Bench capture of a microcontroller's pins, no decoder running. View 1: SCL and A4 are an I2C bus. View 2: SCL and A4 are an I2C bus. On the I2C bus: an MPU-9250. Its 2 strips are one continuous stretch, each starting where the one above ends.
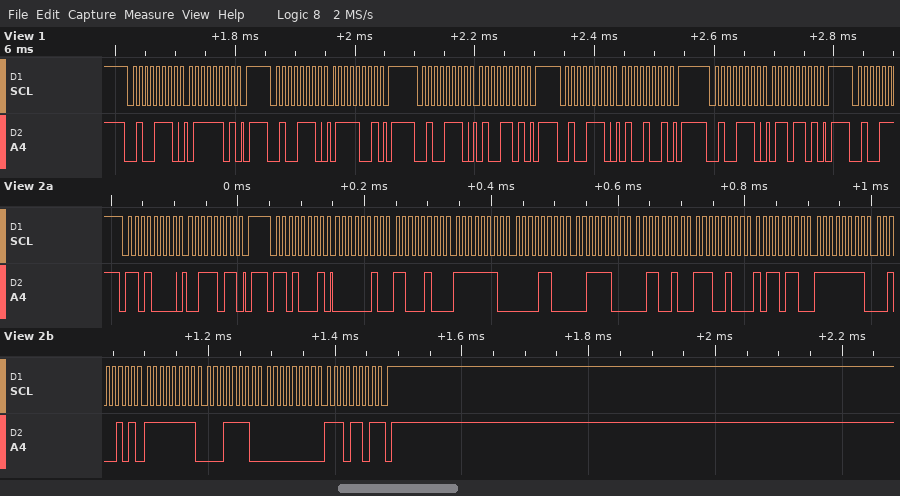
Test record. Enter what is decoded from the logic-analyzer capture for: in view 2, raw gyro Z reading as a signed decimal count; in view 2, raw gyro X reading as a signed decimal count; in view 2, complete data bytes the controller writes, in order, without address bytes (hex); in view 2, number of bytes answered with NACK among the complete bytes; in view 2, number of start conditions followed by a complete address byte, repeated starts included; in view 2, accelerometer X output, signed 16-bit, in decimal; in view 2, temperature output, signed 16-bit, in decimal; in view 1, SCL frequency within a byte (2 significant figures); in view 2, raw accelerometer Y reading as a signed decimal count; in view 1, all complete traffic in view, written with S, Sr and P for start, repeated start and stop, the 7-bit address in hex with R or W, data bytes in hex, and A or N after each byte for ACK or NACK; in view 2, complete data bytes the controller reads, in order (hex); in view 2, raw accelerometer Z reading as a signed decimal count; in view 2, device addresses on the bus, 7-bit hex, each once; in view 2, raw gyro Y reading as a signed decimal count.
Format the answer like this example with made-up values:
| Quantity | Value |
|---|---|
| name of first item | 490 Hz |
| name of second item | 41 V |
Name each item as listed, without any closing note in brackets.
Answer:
| Quantity | Value |
|---|---|
| in view 2, raw gyro Z reading as a signed decimal count | 237 |
| in view 2, raw gyro X reading as a signed decimal count | -219 |
| in view 2, complete data bytes the controller writes, in order, without address bytes | 3B |
| in view 2, number of bytes answered with NACK among the complete bytes | 1 |
| in view 2, number of start conditions followed by a complete address byte, repeated starts included | 2 |
| in view 2, accelerometer X output, signed 16-bit, in decimal | 708 |
| in view 2, temperature output, signed 16-bit, in decimal | -6986 |
| in view 1, SCL frequency within a byte | 100 kHz |
| in view 2, raw accelerometer Y reading as a signed decimal count | -500 |
| in view 1, all complete traffic in view, written with S, Sr and P for start, repeated start and stop, the 7-bit address in hex with R or W, data bytes in hex, and A or N after each byte for ACK or NACK | S 27W A 7D A P S 27W A 79 A P S 27W A 4D A P S 27W A 49 A P S 27W A 6D A P |
| in view 2, complete data bytes the controller reads, in order | 02 C4 FE 0C 3C 32 E4 B6 FF 25 FF 1E 00 ED |
| in view 2, raw accelerometer Z reading as a signed decimal count | 15410 |
| in view 2, device addresses on the bus, 7-bit hex, each once | 0x68 |
| in view 2, raw gyro Y reading as a signed decimal count | -226 |
